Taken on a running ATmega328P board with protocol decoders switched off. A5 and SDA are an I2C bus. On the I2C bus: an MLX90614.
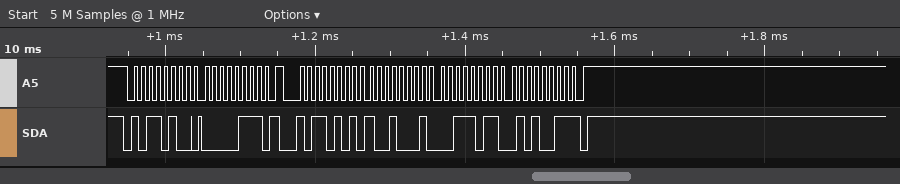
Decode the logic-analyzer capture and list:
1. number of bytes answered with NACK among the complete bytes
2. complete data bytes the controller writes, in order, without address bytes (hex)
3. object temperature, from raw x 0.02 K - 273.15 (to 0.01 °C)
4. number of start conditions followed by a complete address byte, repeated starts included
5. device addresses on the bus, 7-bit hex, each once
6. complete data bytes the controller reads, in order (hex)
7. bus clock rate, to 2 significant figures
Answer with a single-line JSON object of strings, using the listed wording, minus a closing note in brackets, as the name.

{"number of bytes answered with NACK among the complete bytes": "1", "complete data bytes the controller writes, in order, without address bytes": "07", "object temperature, from raw x 0.02 K - 273.15": "31.83 °C", "number of start conditions followed by a complete address byte, repeated starts included": "2", "device addresses on the bus, 7-bit hex, each once": "0x5A", "complete data bytes the controller reads, in order": "91 3B 53", "bus clock rate, to 2 significant figures": "100 kHz"}
